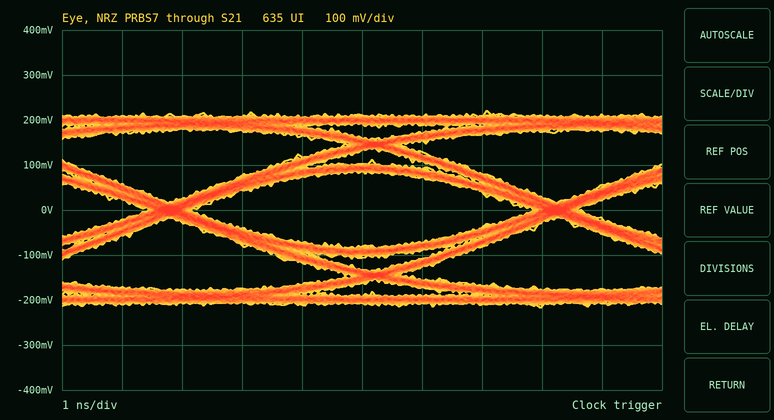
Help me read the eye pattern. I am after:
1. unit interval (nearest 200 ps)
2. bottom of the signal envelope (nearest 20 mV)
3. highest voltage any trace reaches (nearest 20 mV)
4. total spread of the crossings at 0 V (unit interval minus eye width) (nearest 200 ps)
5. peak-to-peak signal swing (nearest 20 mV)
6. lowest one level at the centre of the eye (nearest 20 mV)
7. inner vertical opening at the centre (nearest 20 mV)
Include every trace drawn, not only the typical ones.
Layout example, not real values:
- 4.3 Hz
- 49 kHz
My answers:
- 6.4 ns
- -220 mV
- 220 mV
- 800 ps
- 440 mV
- 80 mV
- 160 mV
